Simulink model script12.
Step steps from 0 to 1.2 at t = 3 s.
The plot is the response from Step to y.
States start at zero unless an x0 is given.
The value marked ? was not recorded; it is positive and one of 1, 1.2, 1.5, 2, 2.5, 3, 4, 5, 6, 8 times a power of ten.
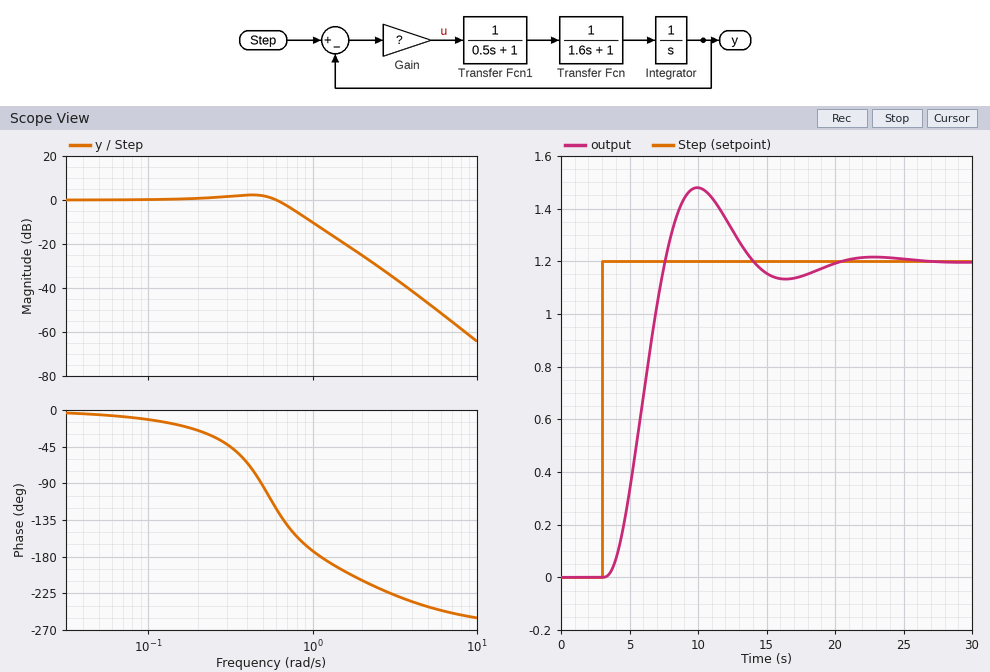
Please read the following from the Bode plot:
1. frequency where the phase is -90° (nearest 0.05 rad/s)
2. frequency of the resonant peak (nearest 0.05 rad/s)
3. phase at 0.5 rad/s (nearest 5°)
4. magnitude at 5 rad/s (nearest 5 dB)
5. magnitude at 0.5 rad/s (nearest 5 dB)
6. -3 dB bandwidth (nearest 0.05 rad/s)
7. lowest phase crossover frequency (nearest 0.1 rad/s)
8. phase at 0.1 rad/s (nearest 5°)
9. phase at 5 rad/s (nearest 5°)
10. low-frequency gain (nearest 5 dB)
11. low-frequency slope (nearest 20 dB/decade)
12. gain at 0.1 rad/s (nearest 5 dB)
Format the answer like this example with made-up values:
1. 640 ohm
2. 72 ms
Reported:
1. 0.50 rad/s
2. 0.40 rad/s
3. -95°
4. -45 dB
5. 0 dB
6. 0.70 rad/s
7. 1.1 rad/s
8. -10°
9. -240°
10. 0 dB
11. 0 dB/decade
12. 0 dB
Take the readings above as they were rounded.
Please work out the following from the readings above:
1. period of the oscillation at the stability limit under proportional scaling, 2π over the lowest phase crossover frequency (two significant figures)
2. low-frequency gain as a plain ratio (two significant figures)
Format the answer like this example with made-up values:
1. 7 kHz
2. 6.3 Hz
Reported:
1. 5.7 s
2. 1.0
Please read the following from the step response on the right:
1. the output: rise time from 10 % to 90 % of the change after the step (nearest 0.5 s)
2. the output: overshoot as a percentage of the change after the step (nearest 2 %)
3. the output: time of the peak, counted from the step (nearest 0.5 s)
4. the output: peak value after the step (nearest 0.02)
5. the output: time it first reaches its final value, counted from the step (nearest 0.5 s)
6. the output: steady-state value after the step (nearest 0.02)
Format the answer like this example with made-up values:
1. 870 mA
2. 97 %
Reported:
1. 3.0 s
2. 24 %
3. 7.0 s
4. 1.48
5. 4.5 s
6. 1.20
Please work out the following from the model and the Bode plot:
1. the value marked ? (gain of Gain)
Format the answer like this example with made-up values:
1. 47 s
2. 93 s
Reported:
1. 0.5
